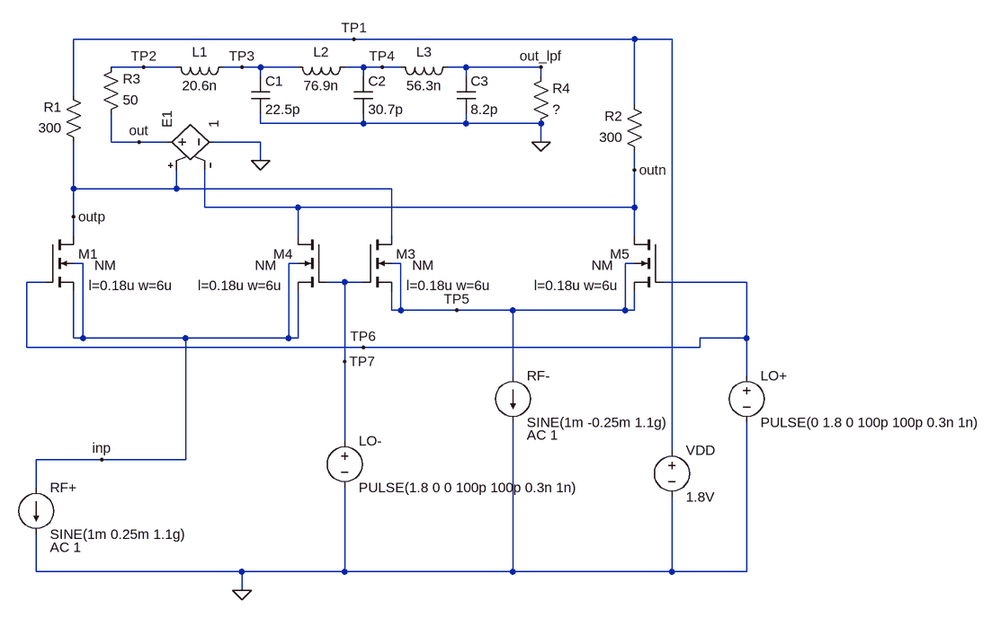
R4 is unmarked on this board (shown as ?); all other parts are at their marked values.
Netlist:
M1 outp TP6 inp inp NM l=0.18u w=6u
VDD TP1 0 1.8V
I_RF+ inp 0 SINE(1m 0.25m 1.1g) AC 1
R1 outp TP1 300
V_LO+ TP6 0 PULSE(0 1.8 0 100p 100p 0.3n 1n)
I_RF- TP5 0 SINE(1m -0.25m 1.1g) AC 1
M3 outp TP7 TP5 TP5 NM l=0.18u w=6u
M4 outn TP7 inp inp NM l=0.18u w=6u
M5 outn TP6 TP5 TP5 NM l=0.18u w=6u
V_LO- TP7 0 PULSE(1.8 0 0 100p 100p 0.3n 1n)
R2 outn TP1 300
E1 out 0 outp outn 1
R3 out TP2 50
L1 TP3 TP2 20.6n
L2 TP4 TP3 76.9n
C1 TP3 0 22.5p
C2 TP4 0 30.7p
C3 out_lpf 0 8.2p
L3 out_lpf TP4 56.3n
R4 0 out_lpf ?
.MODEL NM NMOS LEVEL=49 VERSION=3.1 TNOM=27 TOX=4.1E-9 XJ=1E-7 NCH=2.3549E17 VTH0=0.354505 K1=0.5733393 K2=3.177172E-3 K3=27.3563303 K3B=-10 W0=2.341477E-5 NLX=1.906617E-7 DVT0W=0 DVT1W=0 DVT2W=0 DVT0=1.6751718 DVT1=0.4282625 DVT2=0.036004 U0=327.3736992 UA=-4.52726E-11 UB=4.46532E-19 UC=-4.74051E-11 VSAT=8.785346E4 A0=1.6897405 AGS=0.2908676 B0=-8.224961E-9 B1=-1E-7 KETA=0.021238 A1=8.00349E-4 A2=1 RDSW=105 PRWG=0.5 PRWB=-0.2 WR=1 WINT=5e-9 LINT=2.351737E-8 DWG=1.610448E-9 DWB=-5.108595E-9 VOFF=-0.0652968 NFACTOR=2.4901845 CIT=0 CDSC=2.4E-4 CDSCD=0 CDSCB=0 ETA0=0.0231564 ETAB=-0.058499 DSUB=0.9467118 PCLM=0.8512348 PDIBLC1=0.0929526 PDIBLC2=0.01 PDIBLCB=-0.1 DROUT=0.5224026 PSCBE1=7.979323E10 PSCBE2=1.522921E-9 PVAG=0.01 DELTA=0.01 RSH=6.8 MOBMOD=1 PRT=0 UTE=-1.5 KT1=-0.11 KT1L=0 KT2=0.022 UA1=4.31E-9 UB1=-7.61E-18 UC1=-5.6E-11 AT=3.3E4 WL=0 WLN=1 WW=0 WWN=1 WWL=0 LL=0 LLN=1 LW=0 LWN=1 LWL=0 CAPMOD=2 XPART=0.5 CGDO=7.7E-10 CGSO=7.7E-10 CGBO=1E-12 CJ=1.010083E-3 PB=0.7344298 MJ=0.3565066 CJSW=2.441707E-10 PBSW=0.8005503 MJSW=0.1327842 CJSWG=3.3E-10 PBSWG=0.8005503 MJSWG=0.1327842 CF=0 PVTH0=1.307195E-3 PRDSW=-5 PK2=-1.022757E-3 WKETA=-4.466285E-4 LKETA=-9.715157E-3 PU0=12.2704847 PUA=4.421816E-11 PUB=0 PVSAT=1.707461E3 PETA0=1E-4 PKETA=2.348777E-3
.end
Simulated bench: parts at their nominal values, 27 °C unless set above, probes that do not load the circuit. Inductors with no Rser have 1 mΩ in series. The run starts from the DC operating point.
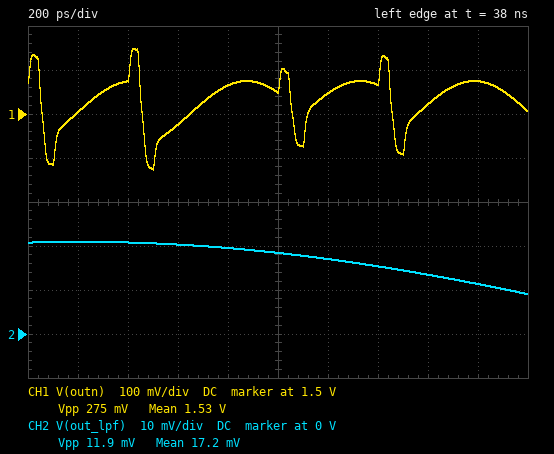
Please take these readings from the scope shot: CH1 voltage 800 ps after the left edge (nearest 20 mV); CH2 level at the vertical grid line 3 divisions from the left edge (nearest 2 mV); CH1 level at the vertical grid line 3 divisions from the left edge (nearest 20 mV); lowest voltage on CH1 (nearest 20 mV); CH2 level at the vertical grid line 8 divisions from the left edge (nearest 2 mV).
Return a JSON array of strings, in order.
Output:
["1.56 V", "20 mV", "1.48 V", "1.38 V", "14 mV"]
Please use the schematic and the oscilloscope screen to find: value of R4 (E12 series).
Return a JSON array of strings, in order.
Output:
["15 Ω"]
